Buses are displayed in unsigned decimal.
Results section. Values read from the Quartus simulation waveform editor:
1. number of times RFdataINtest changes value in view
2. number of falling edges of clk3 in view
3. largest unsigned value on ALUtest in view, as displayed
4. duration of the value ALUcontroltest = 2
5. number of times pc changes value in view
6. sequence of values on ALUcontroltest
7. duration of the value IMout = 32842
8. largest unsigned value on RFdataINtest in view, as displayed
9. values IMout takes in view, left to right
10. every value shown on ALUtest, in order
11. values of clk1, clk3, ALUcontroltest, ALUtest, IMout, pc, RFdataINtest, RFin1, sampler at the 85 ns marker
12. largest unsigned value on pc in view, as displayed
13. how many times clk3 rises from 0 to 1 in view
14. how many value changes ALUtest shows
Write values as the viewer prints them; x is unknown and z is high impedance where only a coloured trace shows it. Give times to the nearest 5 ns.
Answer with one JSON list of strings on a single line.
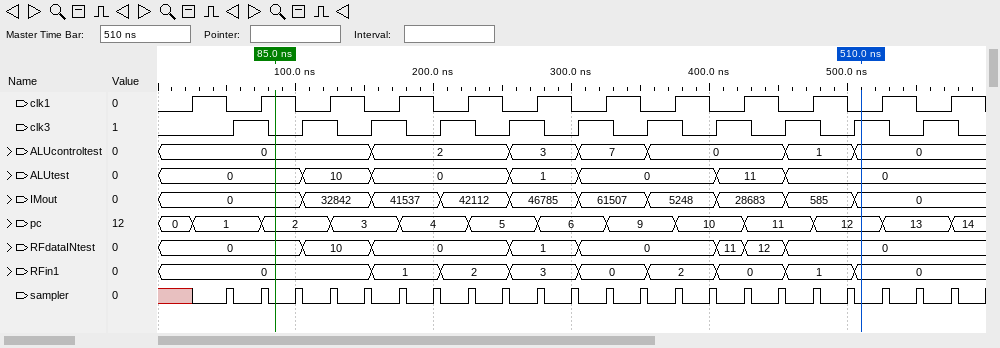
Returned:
["7", "11", "11", "100 ns", "12", "0, 2, 3, 7, 0, 1, 0", "50 ns", "12", "0, 32842, 41537, 42112, 46785, 61507, 5248, 28683, 585, 0", "0, 10, 0, 1, 0, 11, 0", "clk1=1, clk3=0, ALUcontroltest=0, ALUtest=0, IMout=0, pc=2, RFdataINtest=0, RFin1=0, sampler=0", "14", "11", "6"]
